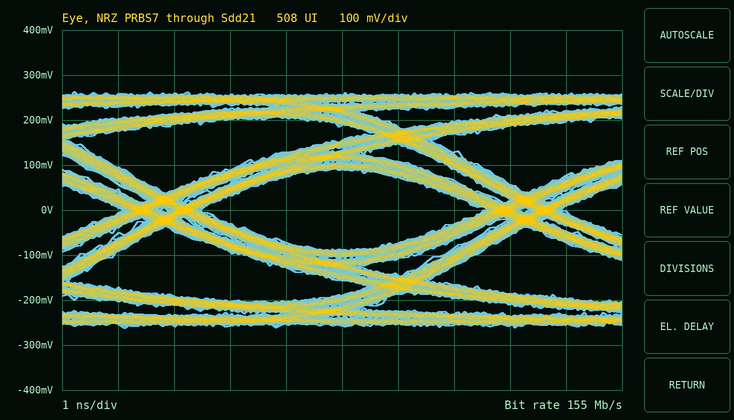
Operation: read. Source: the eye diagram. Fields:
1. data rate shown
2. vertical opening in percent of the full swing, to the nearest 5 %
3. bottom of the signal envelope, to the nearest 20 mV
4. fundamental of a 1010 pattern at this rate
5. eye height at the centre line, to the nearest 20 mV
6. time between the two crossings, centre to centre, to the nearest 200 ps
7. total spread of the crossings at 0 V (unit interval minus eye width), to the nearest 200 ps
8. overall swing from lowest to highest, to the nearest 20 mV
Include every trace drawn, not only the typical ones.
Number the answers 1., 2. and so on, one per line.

1. 155 Mb/s
2. 35 %
3. -260 mV
4. 77.5 MHz
5. 180 mV
6. 6.4 ns
7. 1.4 ns
8. 520 mV
